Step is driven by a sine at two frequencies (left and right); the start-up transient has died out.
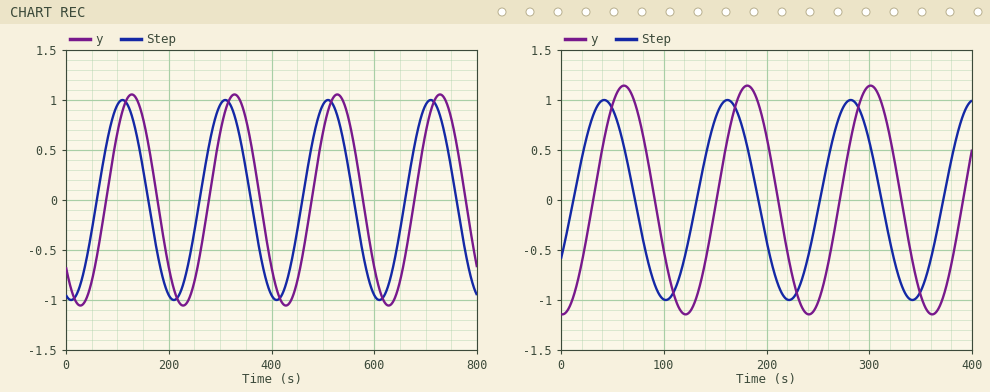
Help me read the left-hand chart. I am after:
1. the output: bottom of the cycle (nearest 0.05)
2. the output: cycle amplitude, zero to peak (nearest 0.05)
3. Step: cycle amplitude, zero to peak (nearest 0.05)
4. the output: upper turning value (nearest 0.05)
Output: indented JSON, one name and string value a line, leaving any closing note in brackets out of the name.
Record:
{
  "the output: bottom of the cycle": "-1.05",
  "the output: cycle amplitude, zero to peak": "1.05",
  "Step: cycle amplitude, zero to peak": "1.00",
  "the output: upper turning value": "1.05"
}
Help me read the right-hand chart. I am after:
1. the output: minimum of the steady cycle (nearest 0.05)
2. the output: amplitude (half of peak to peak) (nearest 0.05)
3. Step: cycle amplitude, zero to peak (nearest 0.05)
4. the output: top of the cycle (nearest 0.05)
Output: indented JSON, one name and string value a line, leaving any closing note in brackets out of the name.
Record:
{
  "the output: minimum of the steady cycle": "-1.15",
  "the output: amplitude (half of peak to peak)": "1.15",
  "Step: cycle amplitude, zero to peak": "1.00",
  "the output: top of the cycle": "1.15"
}
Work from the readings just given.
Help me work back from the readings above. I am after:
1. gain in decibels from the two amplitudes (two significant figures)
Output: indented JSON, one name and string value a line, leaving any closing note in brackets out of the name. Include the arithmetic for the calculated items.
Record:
{
  "gain in decibels from the two amplitudes": "20 log10(1.15 / 1) = 1.2 dB"
}
